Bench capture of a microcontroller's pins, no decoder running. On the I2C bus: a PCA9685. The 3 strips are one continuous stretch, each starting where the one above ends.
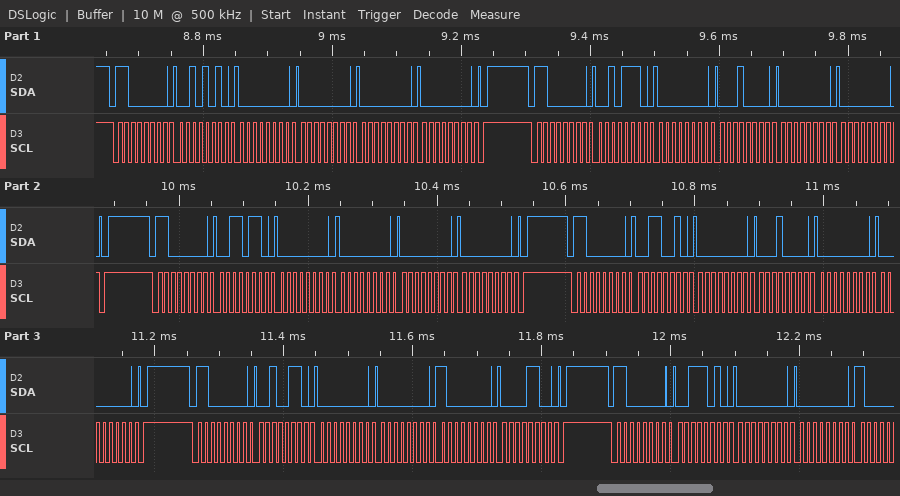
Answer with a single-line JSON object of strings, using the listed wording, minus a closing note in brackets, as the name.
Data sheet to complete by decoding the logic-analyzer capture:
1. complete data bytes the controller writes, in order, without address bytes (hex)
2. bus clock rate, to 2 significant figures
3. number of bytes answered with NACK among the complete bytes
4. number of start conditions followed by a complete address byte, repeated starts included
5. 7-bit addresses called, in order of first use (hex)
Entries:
{"complete data bytes the controller writes, in order, without address bytes": "2A 00 00 00 00 2E 00 10 00 00 36 00 00 00 00 32 00 10 00 00 26 00 00 80 0C 3A 00 00", "bus clock rate, to 2 significant figures": "100 kHz", "number of bytes answered with NACK among the complete bytes": "0", "number of start conditions followed by a complete address byte, repeated starts included": "6", "7-bit addresses called, in order of first use": "0x60"}
